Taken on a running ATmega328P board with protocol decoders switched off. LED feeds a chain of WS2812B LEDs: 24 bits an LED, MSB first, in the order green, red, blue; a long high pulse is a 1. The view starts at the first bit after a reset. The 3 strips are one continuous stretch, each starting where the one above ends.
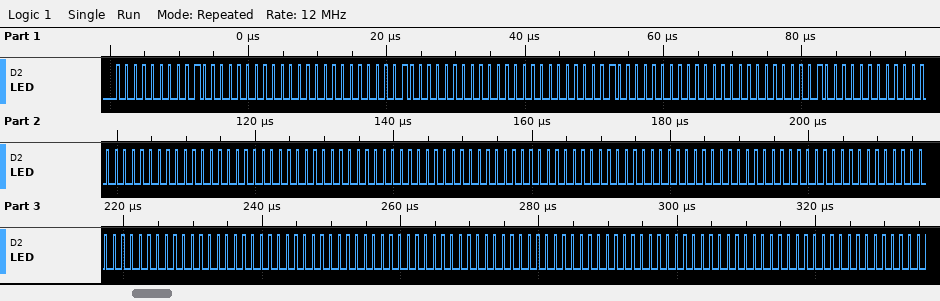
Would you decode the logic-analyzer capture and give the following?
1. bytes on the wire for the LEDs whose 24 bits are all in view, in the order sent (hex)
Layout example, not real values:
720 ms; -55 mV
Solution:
00 40 00 00 40 00 00 40 00 00 40 00 00 00 00 00 00 00 00 00 00 00 00 00 00 00 00 00 00 00 00 00 00
